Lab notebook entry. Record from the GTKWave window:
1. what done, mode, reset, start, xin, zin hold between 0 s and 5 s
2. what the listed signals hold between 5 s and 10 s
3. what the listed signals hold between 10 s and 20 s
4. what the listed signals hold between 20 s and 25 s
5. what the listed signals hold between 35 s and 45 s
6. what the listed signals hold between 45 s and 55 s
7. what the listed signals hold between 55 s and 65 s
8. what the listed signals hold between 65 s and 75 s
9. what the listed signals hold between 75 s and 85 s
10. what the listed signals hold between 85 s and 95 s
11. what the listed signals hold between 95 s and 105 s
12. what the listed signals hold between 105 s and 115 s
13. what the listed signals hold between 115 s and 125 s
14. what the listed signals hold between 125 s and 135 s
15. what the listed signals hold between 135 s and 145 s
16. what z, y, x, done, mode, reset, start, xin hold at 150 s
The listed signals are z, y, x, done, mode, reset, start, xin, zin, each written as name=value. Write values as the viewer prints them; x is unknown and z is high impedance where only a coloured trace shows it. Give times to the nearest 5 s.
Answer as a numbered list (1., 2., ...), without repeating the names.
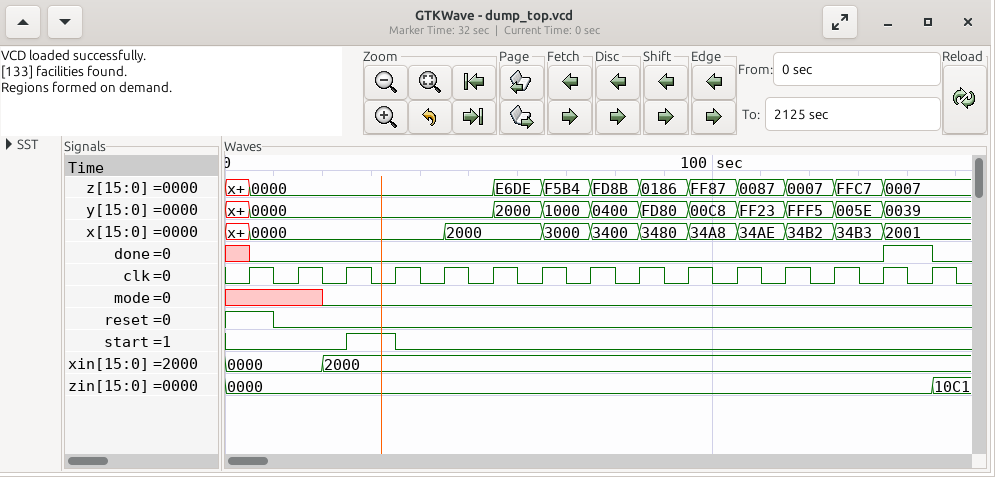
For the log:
1. done=x, mode=x, reset=1, start=0, xin=0000, zin=0000
2. z=0000, y=0000, x=0000, done=0, mode=x, reset=1, start=0, xin=0000, zin=0000
3. z=0000, y=0000, x=0000, done=0, mode=x, reset=0, start=0, xin=0000, zin=0000
4. z=0000, y=0000, x=0000, done=0, mode=0, reset=0, start=0, xin=2000, zin=0000
5. z=0000, y=0000, x=0000, done=0, mode=0, reset=0, start=0, xin=2000, zin=0000
6. z=0000, y=0000, x=2000, done=0, mode=0, reset=0, start=0, xin=2000, zin=0000
7. z=E6DE, y=2000, x=2000, done=0, mode=0, reset=0, start=0, xin=2000, zin=0000
8. z=F5B4, y=1000, x=3000, done=0, mode=0, reset=0, start=0, xin=2000, zin=0000
9. z=FD8B, y=0400, x=3400, done=0, mode=0, reset=0, start=0, xin=2000, zin=0000
10. z=0186, y=FD80, x=3480, done=0, mode=0, reset=0, start=0, xin=2000, zin=0000
11. z=FF87, y=00C8, x=34A8, done=0, mode=0, reset=0, start=0, xin=2000, zin=0000
12. z=0087, y=FF23, x=34AE, done=0, mode=0, reset=0, start=0, xin=2000, zin=0000
13. z=0007, y=FFF5, x=34B2, done=0, mode=0, reset=0, start=0, xin=2000, zin=0000
14. z=FFC7, y=005E, x=34B3, done=0, mode=0, reset=0, start=0, xin=2000, zin=0000
15. z=0007, y=0039, x=2001, done=1, mode=0, reset=0, start=0, xin=2000, zin=0000
16. z=0007, y=0039, x=2001, done=0, mode=0, reset=0, start=0, xin=2000
